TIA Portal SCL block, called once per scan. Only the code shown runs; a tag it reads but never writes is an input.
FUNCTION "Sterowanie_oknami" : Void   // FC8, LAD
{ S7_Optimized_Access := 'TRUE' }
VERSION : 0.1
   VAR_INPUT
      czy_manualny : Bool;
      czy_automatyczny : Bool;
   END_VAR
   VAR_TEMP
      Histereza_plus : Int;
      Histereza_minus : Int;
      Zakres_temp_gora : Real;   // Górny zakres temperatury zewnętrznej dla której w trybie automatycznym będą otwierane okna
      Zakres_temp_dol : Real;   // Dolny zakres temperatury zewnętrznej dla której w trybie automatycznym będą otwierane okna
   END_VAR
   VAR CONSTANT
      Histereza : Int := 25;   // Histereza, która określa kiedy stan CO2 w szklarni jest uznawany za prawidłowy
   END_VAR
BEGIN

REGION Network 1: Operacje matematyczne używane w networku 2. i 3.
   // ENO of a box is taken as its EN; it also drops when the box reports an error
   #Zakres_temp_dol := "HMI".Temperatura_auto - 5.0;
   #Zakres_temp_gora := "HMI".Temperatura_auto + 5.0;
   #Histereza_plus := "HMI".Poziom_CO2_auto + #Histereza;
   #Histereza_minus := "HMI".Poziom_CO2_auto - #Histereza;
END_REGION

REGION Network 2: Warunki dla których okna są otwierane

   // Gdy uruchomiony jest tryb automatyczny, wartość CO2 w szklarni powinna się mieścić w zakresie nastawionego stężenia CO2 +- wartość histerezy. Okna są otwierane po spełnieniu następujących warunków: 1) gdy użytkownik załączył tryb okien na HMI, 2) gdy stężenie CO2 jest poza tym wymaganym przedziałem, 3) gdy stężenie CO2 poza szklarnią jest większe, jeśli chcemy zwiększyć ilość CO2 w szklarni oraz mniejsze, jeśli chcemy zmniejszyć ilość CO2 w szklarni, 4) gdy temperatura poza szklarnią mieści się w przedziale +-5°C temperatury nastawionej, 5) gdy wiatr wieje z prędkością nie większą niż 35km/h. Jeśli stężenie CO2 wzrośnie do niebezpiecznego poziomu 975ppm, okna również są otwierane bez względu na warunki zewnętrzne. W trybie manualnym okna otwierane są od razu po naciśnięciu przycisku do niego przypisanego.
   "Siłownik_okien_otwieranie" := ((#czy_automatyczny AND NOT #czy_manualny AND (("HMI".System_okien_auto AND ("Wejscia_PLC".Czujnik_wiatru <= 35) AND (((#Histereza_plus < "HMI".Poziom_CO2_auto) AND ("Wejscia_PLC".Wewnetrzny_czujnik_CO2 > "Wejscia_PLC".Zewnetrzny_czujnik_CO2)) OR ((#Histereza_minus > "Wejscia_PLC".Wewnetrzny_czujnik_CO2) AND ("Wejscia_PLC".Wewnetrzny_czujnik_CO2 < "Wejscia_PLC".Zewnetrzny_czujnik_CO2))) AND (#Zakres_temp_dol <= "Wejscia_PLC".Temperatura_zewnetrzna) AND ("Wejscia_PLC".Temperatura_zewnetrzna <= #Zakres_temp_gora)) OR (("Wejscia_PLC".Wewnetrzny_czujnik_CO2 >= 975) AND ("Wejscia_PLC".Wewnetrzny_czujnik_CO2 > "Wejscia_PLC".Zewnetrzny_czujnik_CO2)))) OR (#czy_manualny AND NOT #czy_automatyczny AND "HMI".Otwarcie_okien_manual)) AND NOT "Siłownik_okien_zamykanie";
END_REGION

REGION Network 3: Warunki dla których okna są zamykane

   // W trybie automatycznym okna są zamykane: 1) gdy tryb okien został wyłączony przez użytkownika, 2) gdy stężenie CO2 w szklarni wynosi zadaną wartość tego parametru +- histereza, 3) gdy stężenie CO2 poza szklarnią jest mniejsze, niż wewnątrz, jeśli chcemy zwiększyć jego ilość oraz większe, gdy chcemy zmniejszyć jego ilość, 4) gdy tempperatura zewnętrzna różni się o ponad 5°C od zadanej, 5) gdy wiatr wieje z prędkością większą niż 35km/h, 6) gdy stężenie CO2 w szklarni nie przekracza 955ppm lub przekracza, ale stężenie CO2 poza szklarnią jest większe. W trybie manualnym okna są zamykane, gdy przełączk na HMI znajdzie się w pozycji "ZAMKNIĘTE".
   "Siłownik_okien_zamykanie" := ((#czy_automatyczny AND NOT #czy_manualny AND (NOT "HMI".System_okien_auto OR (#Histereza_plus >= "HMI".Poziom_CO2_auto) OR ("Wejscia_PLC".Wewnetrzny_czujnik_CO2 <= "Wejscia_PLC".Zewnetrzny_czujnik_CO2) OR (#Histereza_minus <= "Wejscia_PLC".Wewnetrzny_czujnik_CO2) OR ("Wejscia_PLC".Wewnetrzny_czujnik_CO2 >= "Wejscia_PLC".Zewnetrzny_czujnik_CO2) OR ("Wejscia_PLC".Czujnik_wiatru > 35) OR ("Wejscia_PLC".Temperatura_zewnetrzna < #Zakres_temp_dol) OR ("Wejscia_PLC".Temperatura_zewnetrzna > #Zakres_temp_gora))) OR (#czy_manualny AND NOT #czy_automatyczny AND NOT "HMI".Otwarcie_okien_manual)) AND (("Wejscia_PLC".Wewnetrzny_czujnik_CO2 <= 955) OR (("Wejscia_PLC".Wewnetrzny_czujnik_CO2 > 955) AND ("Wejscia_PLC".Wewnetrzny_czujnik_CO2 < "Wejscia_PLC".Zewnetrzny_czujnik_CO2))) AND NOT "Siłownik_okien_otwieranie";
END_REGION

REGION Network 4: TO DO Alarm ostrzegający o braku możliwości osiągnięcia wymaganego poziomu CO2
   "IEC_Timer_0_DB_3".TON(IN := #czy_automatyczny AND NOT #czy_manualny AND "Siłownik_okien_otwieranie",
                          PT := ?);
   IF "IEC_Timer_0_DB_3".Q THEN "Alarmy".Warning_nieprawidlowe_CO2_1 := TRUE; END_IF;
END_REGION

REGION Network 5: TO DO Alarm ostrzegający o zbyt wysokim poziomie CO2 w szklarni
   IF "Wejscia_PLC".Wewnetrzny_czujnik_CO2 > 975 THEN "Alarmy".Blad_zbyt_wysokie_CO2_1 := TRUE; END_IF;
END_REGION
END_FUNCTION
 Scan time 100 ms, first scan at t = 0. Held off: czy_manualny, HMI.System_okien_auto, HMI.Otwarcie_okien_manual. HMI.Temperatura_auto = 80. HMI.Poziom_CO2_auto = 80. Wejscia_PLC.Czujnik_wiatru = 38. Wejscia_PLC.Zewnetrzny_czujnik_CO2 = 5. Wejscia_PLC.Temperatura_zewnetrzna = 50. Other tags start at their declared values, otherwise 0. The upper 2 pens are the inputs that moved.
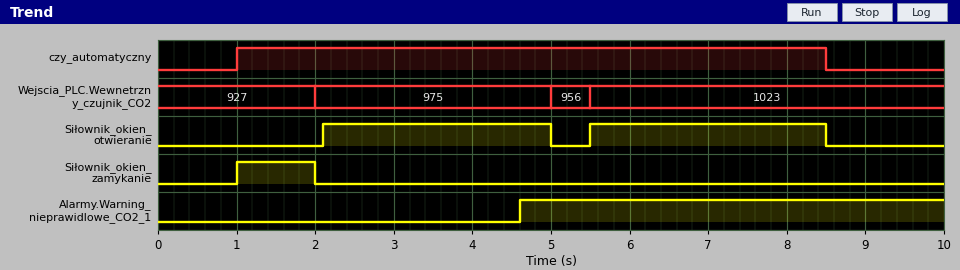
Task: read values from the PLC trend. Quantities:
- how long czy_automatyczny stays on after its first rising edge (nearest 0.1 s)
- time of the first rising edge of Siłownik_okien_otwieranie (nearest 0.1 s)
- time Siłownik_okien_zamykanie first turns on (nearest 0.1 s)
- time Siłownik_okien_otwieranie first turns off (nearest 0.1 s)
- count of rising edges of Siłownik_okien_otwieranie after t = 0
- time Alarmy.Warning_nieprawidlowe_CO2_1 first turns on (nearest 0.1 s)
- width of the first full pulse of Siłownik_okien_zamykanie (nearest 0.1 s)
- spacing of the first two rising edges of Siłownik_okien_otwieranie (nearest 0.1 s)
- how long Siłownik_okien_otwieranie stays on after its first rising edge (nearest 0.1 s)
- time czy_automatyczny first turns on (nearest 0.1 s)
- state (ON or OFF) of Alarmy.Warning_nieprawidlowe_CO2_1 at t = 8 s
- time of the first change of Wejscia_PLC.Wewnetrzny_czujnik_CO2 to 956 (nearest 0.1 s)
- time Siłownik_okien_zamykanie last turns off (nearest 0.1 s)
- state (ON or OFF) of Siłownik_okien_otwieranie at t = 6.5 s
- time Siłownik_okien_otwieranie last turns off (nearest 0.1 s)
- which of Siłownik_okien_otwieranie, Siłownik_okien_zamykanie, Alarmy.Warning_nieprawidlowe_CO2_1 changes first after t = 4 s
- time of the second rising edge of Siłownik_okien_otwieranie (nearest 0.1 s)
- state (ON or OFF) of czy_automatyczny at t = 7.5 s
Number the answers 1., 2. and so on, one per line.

1. 7.5 s
2. 2.1 s
3. 1.0 s
4. 5.0 s
5. 2
6. 4.6 s
7. 1.0 s
8. 3.4 s
9. 2.9 s
10. 1.0 s
11. ON
12. 5.0 s
13. 2.0 s
14. ON
15. 8.5 s
16. Alarmy.Warning_nieprawidlowe_CO2_1
17. 5.5 s
18. ON
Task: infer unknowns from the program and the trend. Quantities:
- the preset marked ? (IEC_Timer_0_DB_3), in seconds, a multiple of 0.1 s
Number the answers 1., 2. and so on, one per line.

1. 2.5 s
